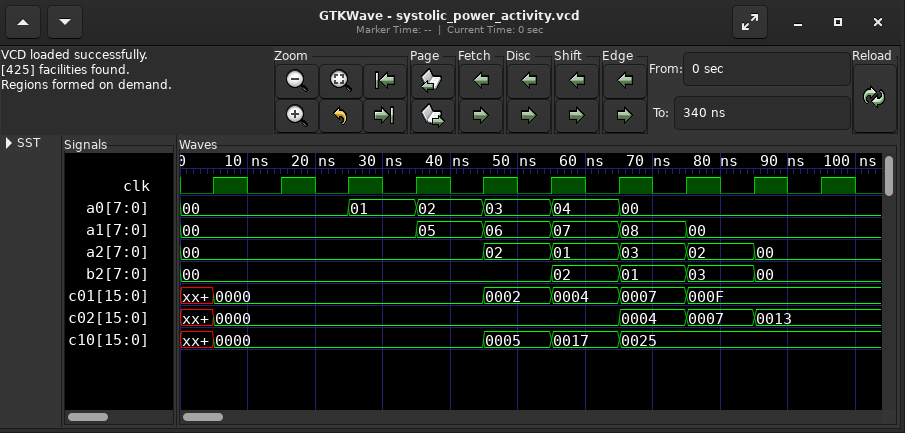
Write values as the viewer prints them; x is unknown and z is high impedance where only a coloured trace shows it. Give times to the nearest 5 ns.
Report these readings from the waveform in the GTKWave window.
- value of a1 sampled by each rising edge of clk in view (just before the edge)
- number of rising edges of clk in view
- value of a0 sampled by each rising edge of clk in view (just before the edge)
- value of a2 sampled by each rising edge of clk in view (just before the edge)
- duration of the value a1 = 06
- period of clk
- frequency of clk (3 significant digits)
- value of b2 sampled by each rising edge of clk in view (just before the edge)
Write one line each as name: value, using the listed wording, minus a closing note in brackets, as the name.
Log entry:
value of a1 sampled by each rising edge of clk in view: 00, 00, 00, 00, 05, 06, 07, 08, 00, 00
number of rising edges of clk in view: 10
value of a0 sampled by each rising edge of clk in view: 00, 00, 00, 01, 02, 03, 04, 00, 00, 00
value of a2 sampled by each rising edge of clk in view: 00, 00, 00, 00, 00, 02, 01, 03, 02, 00
duration of the value a1 = 06: 10 ns
period of clk: 10 ns
frequency of clk: 100 MHz
value of b2 sampled by each rising edge of clk in view: 00, 00, 00, 00, 00, 00, 02, 01, 03, 00
